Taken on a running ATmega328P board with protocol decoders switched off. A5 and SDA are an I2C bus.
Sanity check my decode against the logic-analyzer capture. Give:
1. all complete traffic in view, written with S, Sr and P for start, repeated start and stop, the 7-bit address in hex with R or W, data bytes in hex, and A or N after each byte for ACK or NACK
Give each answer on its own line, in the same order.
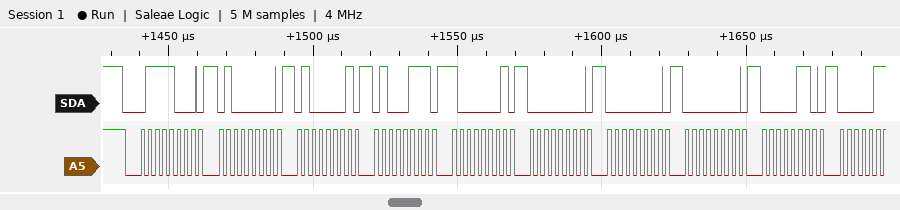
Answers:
S 3CW A 40 A 41 A 47 A 81 A 00 A 00 A 00 A 06 A
